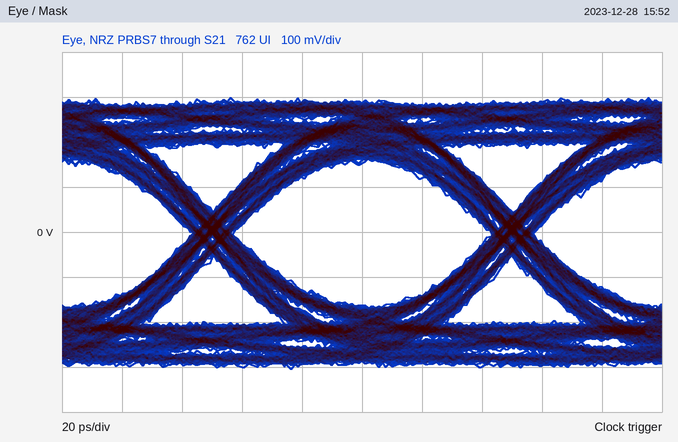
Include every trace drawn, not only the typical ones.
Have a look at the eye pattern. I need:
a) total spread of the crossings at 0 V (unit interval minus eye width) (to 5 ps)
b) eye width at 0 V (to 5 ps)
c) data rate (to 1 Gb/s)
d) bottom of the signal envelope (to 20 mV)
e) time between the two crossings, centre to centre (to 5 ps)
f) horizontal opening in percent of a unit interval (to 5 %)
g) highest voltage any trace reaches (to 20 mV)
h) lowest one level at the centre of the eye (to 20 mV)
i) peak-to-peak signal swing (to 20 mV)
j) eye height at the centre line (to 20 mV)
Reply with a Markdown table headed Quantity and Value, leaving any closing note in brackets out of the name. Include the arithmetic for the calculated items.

| Quantity | Value |
|---|---|
| total spread of the crossings at 0 V (unit interval minus eye width) | 15 ps |
| eye width at 0 V | 85 ps |
| data rate | 10 Gb/s |
| bottom of the signal envelope | -300 mV |
| time between the two crossings, centre to centre | 100 ps |
| horizontal opening in percent of a unit interval | 85 ps / 100 ps ≈ 85 % |
| highest voltage any trace reaches | 300 mV |
| lowest one level at the centre of the eye | 160 mV |
| peak-to-peak signal swing | 600 mV |
| eye height at the centre line | 320 mV |
